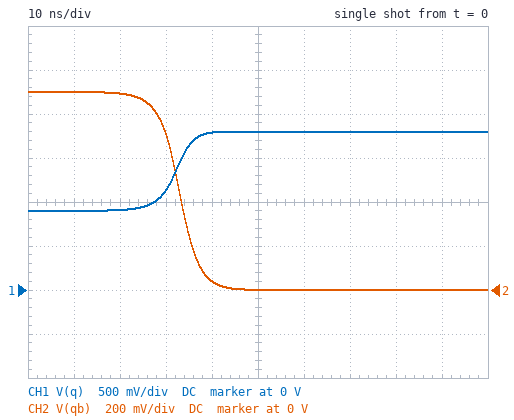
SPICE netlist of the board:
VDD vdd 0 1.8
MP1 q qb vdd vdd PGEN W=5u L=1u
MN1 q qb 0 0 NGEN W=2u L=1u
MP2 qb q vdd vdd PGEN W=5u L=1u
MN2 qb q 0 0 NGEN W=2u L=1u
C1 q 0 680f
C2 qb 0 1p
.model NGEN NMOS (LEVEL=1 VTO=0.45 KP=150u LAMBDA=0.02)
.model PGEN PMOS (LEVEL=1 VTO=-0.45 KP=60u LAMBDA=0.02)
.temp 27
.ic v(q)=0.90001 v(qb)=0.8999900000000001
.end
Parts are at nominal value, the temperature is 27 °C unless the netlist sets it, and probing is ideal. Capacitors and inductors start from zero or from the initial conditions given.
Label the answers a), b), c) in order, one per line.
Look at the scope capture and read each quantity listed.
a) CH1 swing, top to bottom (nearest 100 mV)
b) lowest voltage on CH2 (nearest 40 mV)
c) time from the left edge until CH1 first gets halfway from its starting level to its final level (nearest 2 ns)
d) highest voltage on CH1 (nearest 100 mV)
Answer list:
a) 900 mV
b) 0 V
c) 32 ns
d) 1.8 V
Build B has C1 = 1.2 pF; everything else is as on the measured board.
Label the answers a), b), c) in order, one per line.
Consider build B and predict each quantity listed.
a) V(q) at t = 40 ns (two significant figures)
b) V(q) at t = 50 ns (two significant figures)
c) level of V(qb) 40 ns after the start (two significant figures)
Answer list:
a) 1.1 V
b) 1.7 V
c) 670 mV
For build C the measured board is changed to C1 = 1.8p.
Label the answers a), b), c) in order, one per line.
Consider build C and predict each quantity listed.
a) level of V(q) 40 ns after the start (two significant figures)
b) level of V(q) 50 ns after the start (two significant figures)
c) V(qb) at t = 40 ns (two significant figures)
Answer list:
a) 930 mV
b) 1.1 V
c) 860 mV
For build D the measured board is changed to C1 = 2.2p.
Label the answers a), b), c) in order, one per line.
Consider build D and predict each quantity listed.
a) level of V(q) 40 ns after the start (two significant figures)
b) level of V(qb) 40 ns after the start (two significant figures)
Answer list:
a) 910 mV
b) 880 mV
